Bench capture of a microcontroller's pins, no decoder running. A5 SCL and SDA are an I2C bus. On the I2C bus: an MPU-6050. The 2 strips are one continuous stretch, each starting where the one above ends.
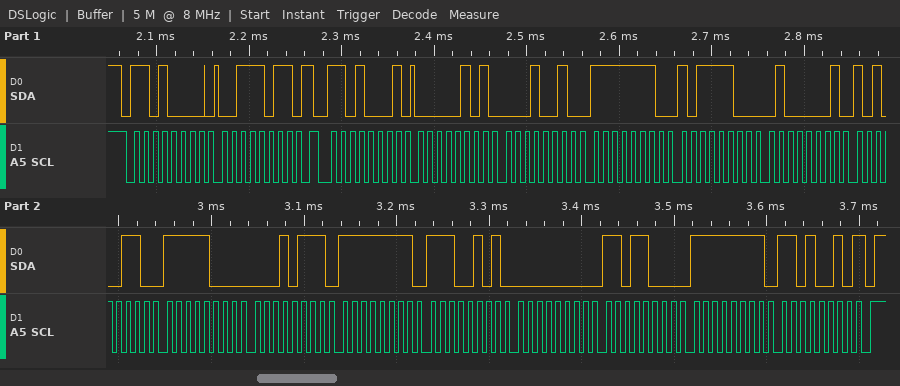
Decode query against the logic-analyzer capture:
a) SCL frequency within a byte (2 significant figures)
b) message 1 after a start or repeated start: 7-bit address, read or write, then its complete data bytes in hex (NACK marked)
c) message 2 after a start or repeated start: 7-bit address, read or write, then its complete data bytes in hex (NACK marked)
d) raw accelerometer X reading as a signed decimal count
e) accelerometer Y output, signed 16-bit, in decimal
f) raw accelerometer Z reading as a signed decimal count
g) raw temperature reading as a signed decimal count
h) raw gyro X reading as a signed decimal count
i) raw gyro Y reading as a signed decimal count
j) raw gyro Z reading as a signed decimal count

100 kHz
0x68 write: 3B
0x68 read: 05 12 FE BC 41 A6 F8 17 FF E5 00 D8 FF D2 NACK
1298
-324
16806
-2025
-27
216
-46
